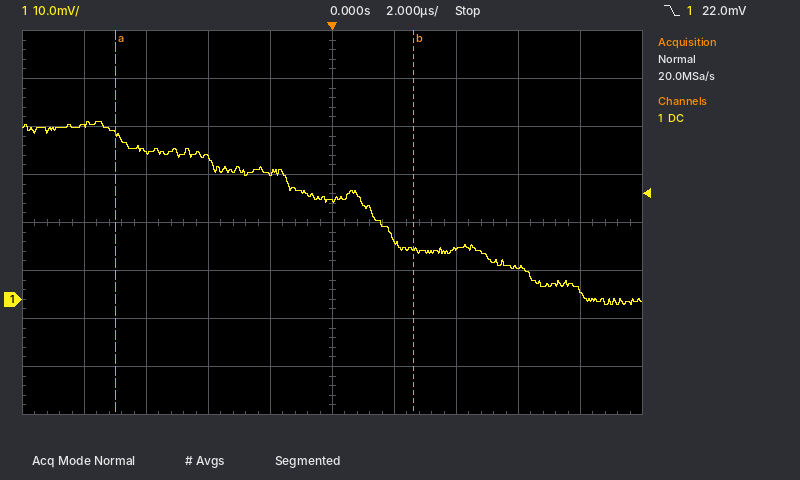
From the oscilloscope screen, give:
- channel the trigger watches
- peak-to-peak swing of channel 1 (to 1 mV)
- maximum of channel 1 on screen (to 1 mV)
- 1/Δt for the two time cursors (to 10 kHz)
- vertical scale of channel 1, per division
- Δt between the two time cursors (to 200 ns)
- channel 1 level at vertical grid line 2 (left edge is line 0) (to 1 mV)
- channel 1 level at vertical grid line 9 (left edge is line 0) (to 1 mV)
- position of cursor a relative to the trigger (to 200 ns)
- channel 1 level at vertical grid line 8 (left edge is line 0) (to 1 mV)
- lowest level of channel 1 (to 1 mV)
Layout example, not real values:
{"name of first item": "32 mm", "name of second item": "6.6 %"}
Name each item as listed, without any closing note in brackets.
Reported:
{"channel the trigger watches": "channel 1", "peak-to-peak swing of channel 1": "38 mV", "maximum of channel 1 on screen": "37 mV", "1/Δt for the two time cursors": "100 kHz", "vertical scale of channel 1, per division": "10 mV", "Δt between the two time cursors": "9.6 µs", "channel 1 level at vertical grid line 2 (left edge is line 0)": "31 mV", "channel 1 level at vertical grid line 9 (left edge is line 0)": "2 mV", "position of cursor a relative to the trigger": "-7.0 µs", "channel 1 level at vertical grid line 8 (left edge is line 0)": "7 mV", "lowest level of channel 1": "-1 mV"}
